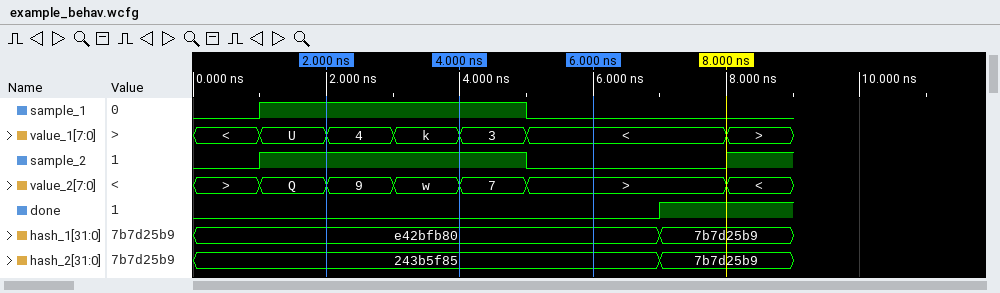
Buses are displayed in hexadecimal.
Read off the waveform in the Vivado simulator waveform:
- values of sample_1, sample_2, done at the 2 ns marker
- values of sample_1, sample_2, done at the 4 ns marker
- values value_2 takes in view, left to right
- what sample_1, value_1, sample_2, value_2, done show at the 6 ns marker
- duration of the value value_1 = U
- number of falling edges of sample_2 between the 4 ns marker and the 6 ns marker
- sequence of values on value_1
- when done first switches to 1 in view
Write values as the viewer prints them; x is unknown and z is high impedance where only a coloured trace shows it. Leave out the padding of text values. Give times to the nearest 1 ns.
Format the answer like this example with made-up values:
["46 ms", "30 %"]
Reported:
["sample_1=1, sample_2=1, done=0", "sample_1=1, sample_2=1, done=0", ">, Q, 9, w, 7, >, <", "sample_1=0, value_1=<, sample_2=0, value_2=>, done=0", "1 ns", "1", "<, U, 4, k, 3, <, >", "7 ns"]
